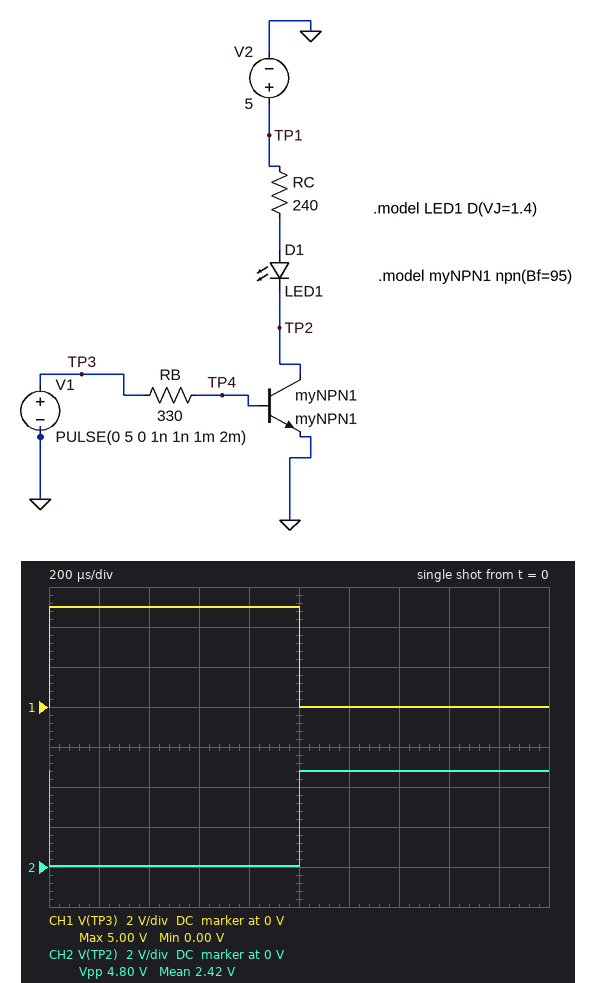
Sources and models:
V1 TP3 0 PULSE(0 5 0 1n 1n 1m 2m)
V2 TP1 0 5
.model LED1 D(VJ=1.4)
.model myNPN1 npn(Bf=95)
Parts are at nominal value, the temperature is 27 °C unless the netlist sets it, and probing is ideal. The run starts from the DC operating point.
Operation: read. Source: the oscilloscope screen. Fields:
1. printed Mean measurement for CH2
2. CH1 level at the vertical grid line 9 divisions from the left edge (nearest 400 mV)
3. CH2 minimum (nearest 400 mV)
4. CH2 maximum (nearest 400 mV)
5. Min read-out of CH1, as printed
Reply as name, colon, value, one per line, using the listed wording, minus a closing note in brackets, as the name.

printed Mean measurement for CH2: 2.42 V
CH1 level at the vertical grid line 9 divisions from the left edge: 0 V
CH2 minimum: 0 V
CH2 maximum: 4.8 V
Min read-out of CH1, as printed: 0.00 V
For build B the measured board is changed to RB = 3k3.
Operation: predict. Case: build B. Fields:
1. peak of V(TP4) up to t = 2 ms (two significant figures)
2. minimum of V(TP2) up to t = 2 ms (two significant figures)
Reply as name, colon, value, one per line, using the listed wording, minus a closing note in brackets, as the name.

peak of V(TP4) up to t = 2 ms: 850 mV
minimum of V(TP2) up to t = 2 ms: 76 mV
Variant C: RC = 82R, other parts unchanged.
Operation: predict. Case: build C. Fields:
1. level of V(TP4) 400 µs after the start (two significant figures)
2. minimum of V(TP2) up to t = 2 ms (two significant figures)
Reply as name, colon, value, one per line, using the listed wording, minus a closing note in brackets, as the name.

level of V(TP4) 400 µs after the start: 890 mV
minimum of V(TP2) up to t = 2 ms: 48 mV
